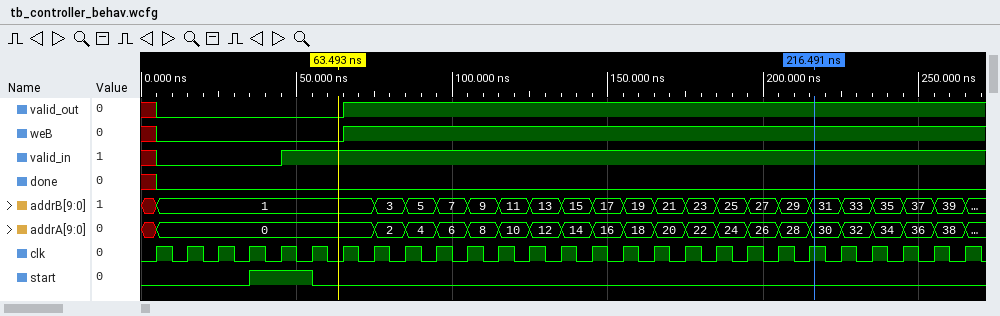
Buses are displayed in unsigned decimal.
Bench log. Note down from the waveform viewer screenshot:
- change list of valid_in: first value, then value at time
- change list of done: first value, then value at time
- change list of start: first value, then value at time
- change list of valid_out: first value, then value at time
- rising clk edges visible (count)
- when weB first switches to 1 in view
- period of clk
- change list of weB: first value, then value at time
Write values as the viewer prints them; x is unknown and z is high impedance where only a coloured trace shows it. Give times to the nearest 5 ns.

x, 0 at 5 ns, 1 at 45 ns
x, 0 at 5 ns
0, 1 at 35 ns, 0 at 55 ns
x, 0 at 5 ns, 1 at 65 ns
27
65 ns
10 ns
x, 0 at 5 ns, 1 at 65 ns
